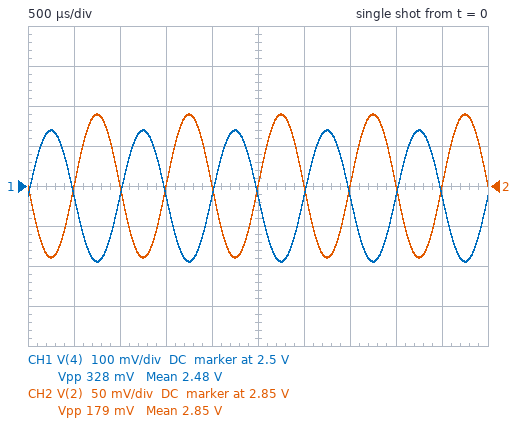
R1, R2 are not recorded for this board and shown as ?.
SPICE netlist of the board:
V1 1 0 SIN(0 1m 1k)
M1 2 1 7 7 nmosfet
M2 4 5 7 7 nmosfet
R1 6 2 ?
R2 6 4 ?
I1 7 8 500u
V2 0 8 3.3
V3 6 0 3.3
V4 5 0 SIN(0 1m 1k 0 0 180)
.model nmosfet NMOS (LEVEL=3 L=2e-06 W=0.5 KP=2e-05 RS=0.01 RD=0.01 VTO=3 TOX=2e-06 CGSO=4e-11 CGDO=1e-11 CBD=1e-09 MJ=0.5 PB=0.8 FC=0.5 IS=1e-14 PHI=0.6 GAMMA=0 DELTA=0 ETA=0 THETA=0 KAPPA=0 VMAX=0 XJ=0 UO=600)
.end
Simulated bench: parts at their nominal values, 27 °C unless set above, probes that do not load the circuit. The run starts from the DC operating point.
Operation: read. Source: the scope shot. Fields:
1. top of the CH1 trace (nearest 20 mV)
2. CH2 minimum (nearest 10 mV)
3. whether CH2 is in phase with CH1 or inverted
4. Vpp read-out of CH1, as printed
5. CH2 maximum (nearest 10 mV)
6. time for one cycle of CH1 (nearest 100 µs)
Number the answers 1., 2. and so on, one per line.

1. 2.64 V
2. 2.76 V
3. inverted
4. 328 mV
5. 2.94 V
6. 1.0 ms
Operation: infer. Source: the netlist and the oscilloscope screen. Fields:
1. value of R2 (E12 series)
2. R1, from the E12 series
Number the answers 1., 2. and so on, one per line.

1. 3.3 kΩ
2. 1.8 kΩ
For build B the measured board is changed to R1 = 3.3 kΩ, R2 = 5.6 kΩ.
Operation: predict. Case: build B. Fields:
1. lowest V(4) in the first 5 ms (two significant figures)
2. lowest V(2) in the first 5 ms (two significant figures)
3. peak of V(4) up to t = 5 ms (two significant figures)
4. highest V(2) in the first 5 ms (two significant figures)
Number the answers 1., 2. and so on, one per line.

1. 1.6 V
2. 2.3 V
3. 2.2 V
4. 2.6 V
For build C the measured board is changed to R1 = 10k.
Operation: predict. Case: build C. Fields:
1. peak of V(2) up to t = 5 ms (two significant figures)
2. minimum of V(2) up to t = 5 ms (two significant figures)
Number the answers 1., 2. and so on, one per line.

1. 1.3 V
2. 300 mV
